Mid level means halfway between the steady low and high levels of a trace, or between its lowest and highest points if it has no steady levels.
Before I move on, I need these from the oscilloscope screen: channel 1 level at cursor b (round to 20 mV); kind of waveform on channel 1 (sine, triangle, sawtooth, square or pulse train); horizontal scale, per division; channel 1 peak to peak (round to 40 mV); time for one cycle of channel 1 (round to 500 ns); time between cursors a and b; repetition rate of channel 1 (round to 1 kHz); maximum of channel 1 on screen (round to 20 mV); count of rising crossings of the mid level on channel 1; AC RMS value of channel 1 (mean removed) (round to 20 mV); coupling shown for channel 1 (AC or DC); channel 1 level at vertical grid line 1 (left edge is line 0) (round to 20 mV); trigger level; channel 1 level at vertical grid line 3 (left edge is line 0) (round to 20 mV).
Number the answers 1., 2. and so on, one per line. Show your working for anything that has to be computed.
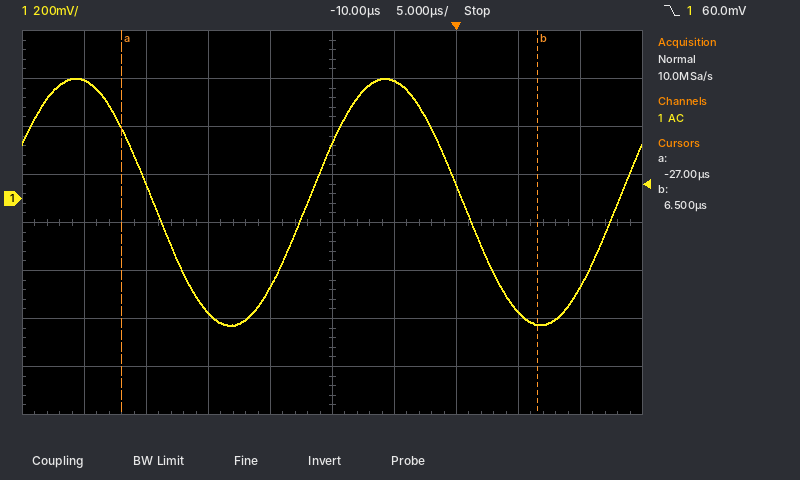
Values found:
1. -520 mV
2. sine
3. 5 µs
4. 1.04 V
5. 25.0 µs
6. 6.5 µs − (-27 µs) = 33.5 µs
7. 1 / 25.0 µs ≈ 40 kHz
8. 500 mV
9. 2
10. 1.04 V / (2√2) ≈ 368 mV, so 360 mV to the nearest 20 mV
11. AC
12. 500 mV
13. 60.0 mV
14. -480 mV
